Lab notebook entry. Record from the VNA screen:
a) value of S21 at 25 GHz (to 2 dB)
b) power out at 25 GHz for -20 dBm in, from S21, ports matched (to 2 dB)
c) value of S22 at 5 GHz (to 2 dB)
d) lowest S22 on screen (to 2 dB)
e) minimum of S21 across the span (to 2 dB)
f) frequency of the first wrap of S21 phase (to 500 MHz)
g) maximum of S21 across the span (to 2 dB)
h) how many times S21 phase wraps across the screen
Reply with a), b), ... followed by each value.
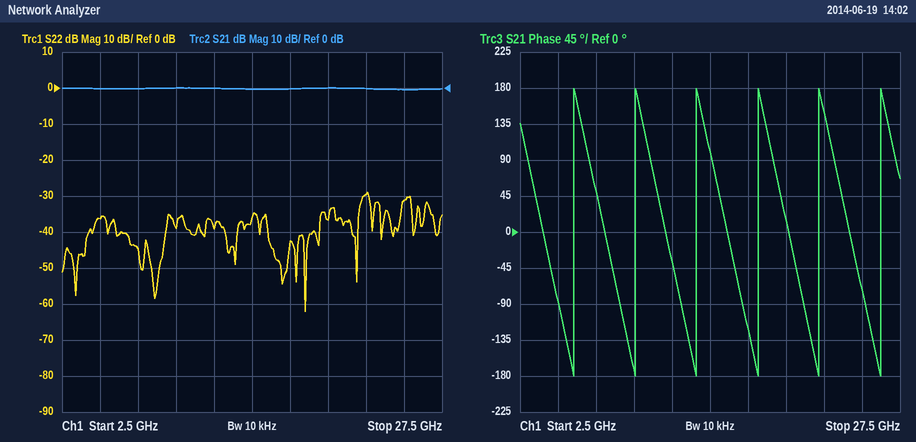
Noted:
a) 0 dB
b) -20 dBm
c) -36 dB
d) -62 dB
e) 0 dB
f) 6.0 GHz
g) 0 dB
h) 6
